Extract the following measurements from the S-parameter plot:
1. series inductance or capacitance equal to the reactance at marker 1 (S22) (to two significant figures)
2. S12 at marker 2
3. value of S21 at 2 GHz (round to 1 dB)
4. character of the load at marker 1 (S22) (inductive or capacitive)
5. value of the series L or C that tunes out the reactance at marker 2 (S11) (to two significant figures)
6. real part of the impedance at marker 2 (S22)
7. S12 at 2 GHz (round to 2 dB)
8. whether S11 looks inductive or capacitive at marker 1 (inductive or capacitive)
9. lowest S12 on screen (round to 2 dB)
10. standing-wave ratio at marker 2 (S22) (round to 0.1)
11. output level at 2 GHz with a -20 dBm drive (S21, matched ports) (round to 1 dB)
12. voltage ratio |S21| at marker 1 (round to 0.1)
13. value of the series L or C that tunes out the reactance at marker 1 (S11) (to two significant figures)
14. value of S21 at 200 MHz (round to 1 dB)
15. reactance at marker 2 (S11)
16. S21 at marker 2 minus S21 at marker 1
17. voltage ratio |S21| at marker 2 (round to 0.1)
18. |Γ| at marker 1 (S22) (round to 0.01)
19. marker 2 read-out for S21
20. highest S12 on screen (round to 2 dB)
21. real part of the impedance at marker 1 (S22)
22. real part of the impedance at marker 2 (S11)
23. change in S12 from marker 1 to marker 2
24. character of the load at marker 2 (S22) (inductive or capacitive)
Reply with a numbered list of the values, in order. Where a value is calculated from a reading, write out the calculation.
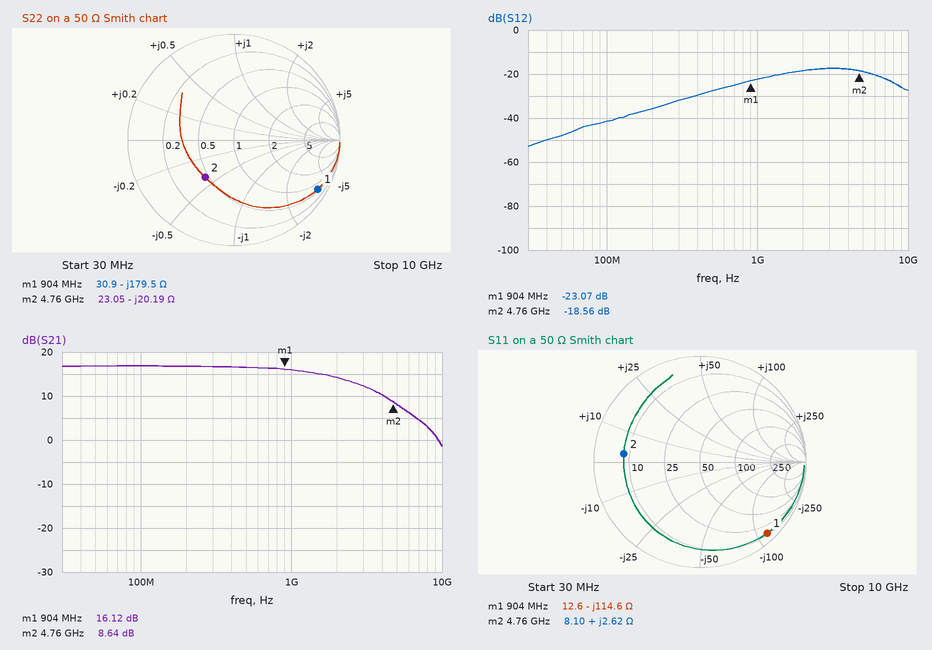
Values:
1. C = 1/(2π × 904 MHz × 179.5 Ω) ≈ 981 fF, so 980 fF to two significant figures
2. -18.56 dB
3. 14 dB
4. capacitive
5. C = 1/(2π × 4.76 GHz × 2.62 Ω) ≈ 13 pF
6. 23.05 Ω
7. -18 dB
8. capacitive
9. -52 dB
10. 2.6
11. -20 dBm + (14 dB) = -6 dBm
12. 10^(16.12/20) ≈ 6.4
13. L = 114.6 Ω/(2π × 904 MHz) ≈ 20 nH
14. 17 dB
15. +2.62 Ω
16. 8.64 − (16.12) = -7.48 dB
17. 10^(8.64/20) ≈ 2.7
18. 0.92
19. 8.64 dB
20. -18 dB
21. 30.9 Ω
22. 8.10 Ω
23. -18.56 − (-23.07) = 4.51 dB
24. capacitive
